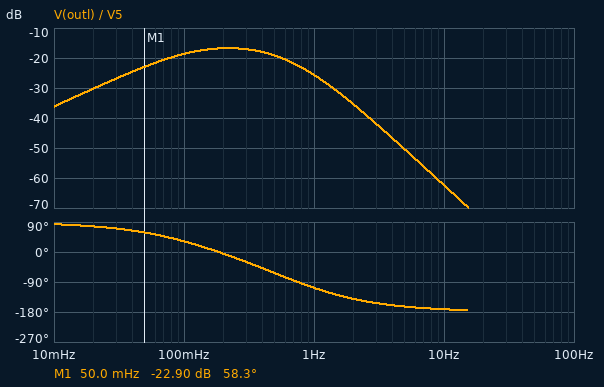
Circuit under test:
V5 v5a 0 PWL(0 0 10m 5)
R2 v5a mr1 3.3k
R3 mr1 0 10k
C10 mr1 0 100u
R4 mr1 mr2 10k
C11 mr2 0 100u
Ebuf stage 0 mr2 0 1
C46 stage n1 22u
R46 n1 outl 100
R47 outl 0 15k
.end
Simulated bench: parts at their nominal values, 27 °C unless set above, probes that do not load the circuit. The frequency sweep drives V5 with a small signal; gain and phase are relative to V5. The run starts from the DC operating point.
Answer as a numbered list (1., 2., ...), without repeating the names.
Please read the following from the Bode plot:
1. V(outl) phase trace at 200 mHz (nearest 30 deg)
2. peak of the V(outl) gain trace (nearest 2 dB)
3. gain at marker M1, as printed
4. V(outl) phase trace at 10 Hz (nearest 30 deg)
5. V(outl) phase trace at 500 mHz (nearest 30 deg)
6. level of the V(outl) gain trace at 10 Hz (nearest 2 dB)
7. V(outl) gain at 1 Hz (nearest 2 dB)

1. 0 deg
2. -16 dB
3. -22.90 dB
4. -180 deg
5. -60 deg
6. -62 dB
7. -26 dB
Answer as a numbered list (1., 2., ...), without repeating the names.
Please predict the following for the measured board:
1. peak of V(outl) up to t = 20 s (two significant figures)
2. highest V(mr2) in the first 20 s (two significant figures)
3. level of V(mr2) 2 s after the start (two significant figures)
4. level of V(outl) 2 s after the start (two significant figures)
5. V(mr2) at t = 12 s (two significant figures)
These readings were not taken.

1. 560 mV
2. 3.8 V
3. 2.8 V
4. 320 mV
5. 3.8 V
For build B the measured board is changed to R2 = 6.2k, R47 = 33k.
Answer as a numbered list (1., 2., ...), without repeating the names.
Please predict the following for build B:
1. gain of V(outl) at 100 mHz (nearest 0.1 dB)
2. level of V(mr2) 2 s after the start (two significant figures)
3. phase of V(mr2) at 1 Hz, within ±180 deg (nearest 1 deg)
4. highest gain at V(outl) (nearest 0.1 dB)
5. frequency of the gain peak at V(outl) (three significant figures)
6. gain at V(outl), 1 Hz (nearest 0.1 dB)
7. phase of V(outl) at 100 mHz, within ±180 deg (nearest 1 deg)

1. -14.7 dB
2. 2.1 V
3. -142 deg
4. -14.2 dB
5. 143 mHz
6. -29.5 dB
7. 13 deg
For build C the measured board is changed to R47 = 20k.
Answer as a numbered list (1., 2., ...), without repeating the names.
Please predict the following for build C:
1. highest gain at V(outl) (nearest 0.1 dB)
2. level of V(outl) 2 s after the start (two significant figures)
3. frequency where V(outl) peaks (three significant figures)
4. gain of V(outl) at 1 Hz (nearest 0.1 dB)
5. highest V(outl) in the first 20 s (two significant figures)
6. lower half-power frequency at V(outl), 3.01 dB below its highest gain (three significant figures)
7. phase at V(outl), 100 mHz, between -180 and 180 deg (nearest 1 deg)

1. -14.7 dB
2. 450 mV
3. 196 mHz
4. -25.2 dB
5. 700 mV
6. 75.5 mHz
7. 28 deg
